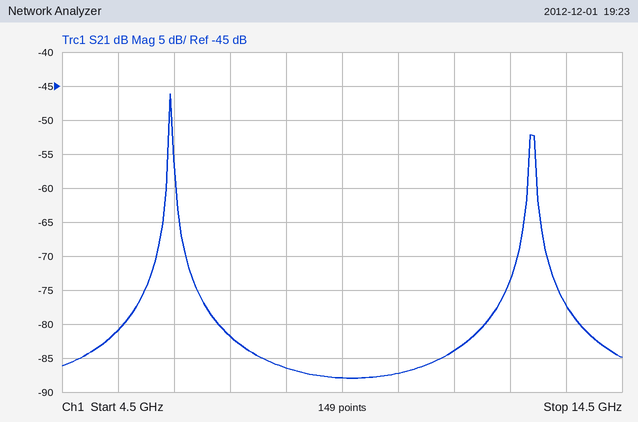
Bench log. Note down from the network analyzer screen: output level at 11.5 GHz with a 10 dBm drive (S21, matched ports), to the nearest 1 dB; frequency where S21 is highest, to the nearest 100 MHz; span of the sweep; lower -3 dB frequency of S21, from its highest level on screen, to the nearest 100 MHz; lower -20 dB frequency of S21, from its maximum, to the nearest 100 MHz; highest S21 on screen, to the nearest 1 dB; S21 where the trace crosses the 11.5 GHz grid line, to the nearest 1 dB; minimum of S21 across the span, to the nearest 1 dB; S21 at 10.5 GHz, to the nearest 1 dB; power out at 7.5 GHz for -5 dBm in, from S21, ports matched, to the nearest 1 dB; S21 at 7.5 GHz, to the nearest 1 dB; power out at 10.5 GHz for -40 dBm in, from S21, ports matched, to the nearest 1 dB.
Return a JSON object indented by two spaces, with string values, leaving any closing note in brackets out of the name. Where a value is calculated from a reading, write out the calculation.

{
  "output level at 11.5 GHz with a 10 dBm drive (S21, matched ports), to the nearest 1 dB": "10 dBm + (-84 dB) = -74 dBm",
  "frequency where S21 is highest, to the nearest 100 MHz": "6.4 GHz",
  "span of the sweep": "10 GHz",
  "lower -3 dB frequency of S21, from its highest level on screen, to the nearest 100 MHz": "6.4 GHz",
  "lower -20 dB frequency of S21, from its maximum, to the nearest 100 MHz": "6.3 GHz",
  "highest S21 on screen, to the nearest 1 dB": "-46 dB",
  "S21 where the trace crosses the 11.5 GHz grid line, to the nearest 1 dB": "-84 dB",
  "minimum of S21 across the span, to the nearest 1 dB": "-88 dB",
  "S21 at 10.5 GHz, to the nearest 1 dB": "-87 dB",
  "power out at 7.5 GHz for -5 dBm in, from S21, ports matched, to the nearest 1 dB": "-5 dBm + (-82 dB) = -87 dBm",
  "S21 at 7.5 GHz, to the nearest 1 dB": "-82 dB",
  "power out at 10.5 GHz for -40 dBm in, from S21, ports matched, to the nearest 1 dB": "-40 dBm + (-87 dB) = -127 dBm"
}
